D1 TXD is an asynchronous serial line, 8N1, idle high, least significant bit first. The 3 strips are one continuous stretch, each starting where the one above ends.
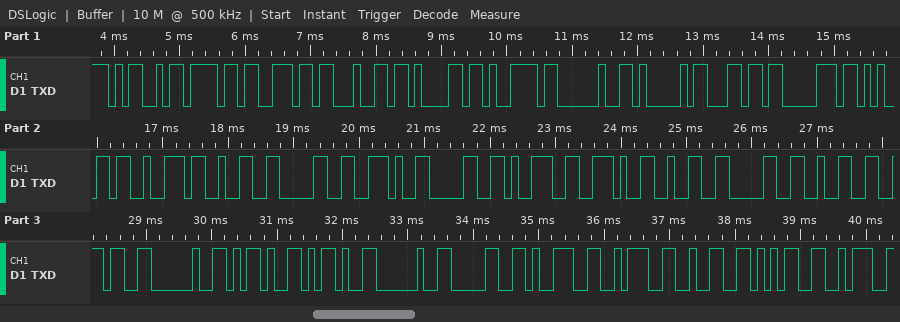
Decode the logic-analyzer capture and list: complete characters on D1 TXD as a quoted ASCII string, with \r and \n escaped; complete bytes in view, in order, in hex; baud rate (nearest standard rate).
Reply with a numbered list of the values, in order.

1. "Monday Alper20.09.2026 -- 09:25:"
2. 4D 6F 6E 64 61 79 20 41 6C 70 65 72 32 30 2E 30 39 2E 32 30 32 36 20 2D 2D 20 30 39 3A 32 35 3A
3. 9600 baud
